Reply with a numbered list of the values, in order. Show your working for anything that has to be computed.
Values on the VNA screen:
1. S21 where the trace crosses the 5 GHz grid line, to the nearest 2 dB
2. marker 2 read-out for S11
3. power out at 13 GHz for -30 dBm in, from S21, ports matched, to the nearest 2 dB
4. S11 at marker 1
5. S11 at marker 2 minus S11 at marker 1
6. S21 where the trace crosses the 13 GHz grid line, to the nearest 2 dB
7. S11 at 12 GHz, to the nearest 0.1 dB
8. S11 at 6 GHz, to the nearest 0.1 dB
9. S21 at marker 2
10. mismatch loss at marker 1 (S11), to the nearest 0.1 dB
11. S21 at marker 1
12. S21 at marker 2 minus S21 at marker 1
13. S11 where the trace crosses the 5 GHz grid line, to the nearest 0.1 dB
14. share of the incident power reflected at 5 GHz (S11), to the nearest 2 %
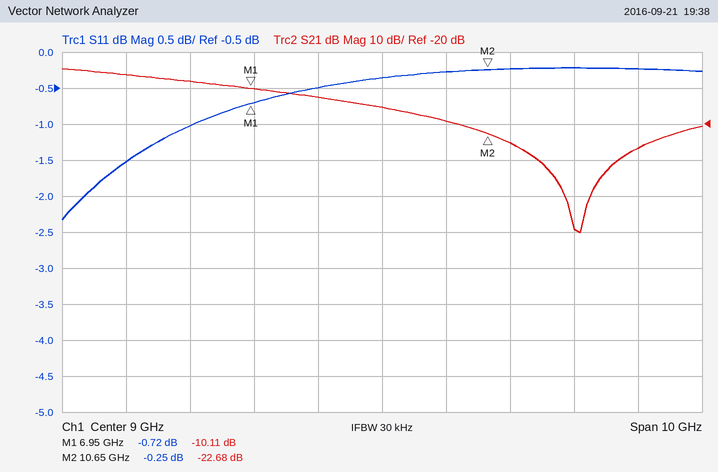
1. -6 dB
2. -0.25 dB
3. -30 dBm + (-26 dB) = -56 dBm
4. -0.72 dB
5. -0.25 − (-0.72) = 0.47 dB
6. -26 dB
7. -0.2 dB
8. -1.0 dB
9. -22.68 dB
10. −10 log10(1 − 10^(-0.72/10)) ≈ 8.2 dB
11. -10.11 dB
12. -22.68 − (-10.11) = -12.57 dB
13. -1.5 dB
14. 10^(-1.5/10) ≈ 70.8 %, so 70 % to the nearest 2 %
